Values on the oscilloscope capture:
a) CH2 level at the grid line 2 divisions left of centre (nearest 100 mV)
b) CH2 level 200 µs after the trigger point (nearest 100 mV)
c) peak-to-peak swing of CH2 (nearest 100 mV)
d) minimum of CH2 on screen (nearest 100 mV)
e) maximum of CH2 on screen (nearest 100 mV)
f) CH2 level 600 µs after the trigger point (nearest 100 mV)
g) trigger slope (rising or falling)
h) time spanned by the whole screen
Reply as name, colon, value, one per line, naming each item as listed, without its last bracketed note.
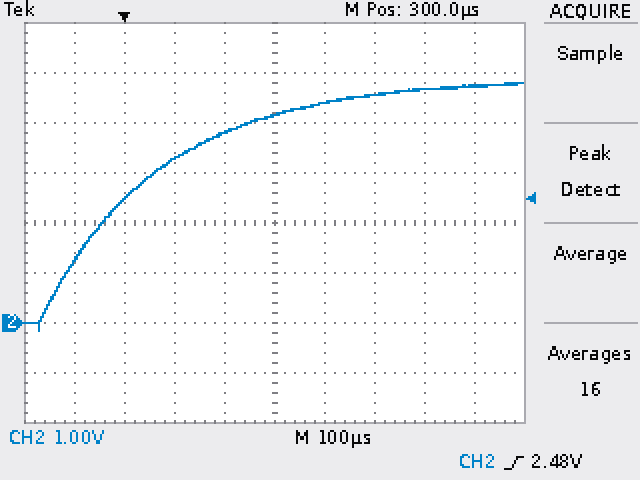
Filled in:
CH2 level at the grid line 2 divisions left of centre: 3.3 V
CH2 level 200 µs after the trigger point: 3.8 V
peak-to-peak swing of CH2: 5.0 V
minimum of CH2 on screen: -200 mV
maximum of CH2 on screen: 4.8 V
CH2 level 600 µs after the trigger point: 4.7 V
trigger slope: rising
time spanned by the whole screen: 1 ms
